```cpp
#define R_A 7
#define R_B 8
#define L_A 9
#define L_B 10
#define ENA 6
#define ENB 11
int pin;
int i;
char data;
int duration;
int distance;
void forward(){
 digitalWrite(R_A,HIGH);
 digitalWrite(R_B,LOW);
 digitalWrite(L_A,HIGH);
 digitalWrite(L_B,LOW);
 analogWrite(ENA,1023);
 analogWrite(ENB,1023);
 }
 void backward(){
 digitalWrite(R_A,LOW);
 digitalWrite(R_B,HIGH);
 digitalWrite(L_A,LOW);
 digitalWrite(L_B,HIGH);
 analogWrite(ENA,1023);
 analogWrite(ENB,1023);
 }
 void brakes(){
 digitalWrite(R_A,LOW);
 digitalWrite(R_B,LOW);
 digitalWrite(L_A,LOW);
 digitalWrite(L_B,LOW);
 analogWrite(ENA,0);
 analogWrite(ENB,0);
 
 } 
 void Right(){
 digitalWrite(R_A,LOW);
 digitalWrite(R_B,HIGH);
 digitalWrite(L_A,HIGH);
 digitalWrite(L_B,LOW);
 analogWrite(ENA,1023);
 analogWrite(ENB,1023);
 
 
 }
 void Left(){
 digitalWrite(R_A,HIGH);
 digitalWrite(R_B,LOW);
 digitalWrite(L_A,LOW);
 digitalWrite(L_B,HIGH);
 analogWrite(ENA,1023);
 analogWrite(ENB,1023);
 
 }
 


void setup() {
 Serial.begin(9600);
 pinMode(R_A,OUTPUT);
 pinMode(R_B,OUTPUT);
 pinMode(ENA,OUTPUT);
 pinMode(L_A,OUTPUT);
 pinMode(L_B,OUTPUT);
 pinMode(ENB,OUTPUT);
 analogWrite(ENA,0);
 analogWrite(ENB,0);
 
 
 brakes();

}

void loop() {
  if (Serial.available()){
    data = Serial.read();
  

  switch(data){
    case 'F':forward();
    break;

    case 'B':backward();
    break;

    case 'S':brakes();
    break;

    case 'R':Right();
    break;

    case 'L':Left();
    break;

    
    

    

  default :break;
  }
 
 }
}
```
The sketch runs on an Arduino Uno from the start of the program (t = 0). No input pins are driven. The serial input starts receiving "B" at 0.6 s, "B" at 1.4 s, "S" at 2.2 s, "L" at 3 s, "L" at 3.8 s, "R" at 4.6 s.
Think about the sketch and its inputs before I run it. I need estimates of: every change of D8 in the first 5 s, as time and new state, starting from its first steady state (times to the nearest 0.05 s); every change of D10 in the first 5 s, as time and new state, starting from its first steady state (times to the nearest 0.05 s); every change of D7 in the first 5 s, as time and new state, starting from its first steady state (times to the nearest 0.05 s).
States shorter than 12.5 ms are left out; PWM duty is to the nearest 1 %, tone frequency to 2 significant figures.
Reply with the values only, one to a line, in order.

0 s low; 0.6 s high; 2.2 s low; 4.6 s high
0 s low; 0.6 s high; 2.2 s low; 3 s high; 4.6 s low
0 s low; 3 s high; 4.6 s low
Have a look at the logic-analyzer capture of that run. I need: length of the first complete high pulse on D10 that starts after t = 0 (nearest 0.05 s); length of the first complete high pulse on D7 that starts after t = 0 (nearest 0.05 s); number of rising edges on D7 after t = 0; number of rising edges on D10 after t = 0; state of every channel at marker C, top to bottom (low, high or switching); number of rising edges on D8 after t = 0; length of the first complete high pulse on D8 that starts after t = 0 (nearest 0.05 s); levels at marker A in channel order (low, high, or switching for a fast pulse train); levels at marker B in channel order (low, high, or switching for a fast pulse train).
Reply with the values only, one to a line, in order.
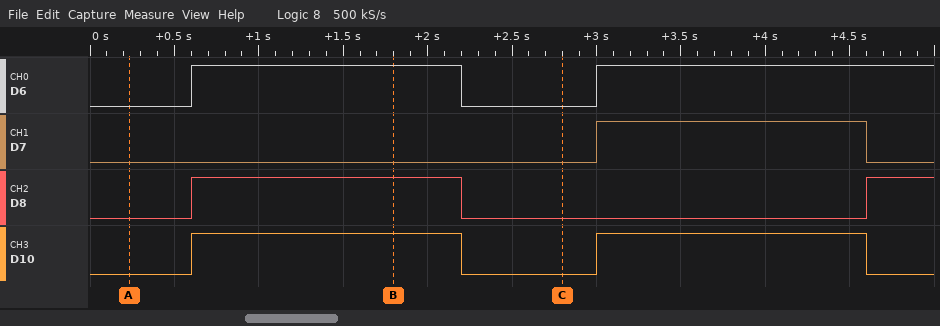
1.60 s
1.60 s
1
2
D6 low, D7 low, D8 low, D10 low
2
1.60 s
D6 low, D7 low, D8 low, D10 low
D6 high, D7 low, D8 high, D10 high
